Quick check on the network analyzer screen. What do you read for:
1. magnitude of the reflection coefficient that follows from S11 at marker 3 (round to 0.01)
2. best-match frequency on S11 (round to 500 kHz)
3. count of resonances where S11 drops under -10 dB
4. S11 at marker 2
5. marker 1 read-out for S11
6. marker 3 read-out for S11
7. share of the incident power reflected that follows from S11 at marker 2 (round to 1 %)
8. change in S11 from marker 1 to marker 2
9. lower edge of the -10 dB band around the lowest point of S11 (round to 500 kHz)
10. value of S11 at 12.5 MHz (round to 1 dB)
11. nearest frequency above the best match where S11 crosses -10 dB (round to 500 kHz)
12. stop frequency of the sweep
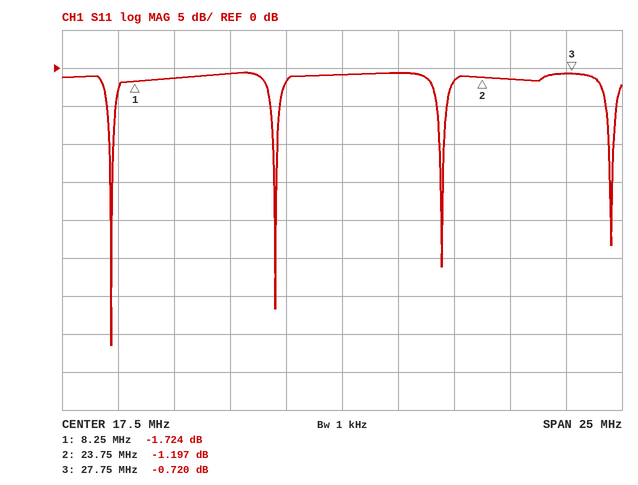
0.92
7.0 MHz
4
-1.197 dB
-1.724 dB
-0.720 dB
76 %
0.527 dB
7.0 MHz
-1 dB
7.5 MHz
30 MHz
